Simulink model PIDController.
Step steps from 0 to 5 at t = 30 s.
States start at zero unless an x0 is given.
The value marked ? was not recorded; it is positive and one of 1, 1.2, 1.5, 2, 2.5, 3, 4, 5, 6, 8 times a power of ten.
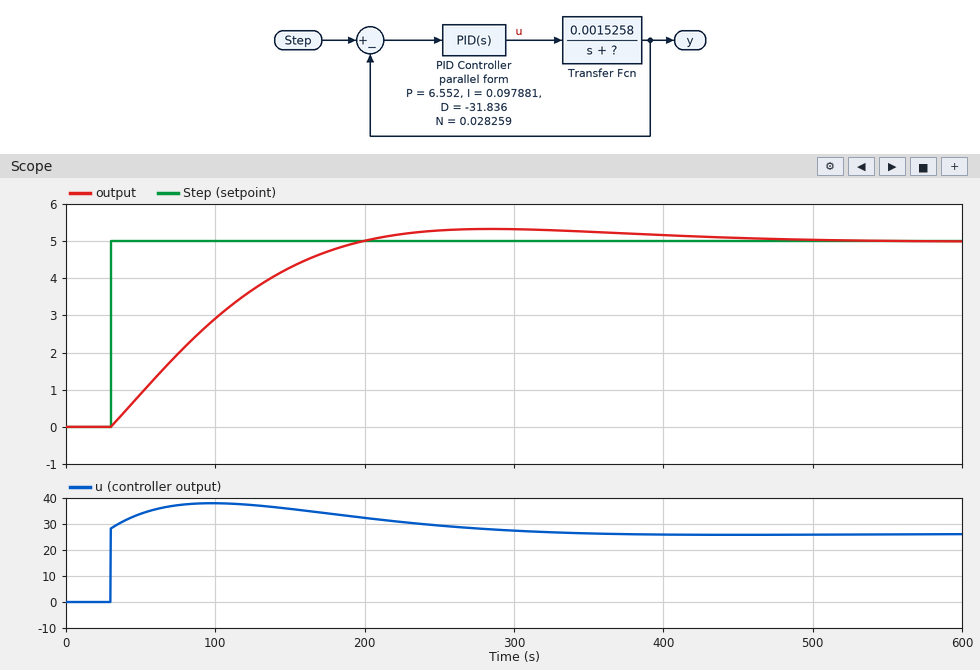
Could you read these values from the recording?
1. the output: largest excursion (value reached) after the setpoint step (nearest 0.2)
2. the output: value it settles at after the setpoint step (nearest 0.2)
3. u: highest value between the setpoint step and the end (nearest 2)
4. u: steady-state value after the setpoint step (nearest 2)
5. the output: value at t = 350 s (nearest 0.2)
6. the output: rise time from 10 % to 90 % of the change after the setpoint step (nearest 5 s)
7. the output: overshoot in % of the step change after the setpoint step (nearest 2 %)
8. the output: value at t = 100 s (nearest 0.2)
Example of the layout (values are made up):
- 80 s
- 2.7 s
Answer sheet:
- 5.4
- 5.0
- 38
- 26
- 5.2
- 120 s
- 6 %
- 3.0
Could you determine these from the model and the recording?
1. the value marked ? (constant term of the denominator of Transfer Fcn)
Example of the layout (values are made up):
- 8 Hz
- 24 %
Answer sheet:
- 0.008
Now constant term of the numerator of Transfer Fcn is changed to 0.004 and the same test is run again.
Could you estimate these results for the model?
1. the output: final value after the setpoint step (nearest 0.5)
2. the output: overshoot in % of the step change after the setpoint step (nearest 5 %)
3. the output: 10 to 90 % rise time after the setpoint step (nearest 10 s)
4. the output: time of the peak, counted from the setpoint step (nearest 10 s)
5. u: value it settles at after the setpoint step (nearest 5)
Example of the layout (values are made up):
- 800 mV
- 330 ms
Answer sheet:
- 5.0
- 10 %
- 60 s
- 130 s
- 10
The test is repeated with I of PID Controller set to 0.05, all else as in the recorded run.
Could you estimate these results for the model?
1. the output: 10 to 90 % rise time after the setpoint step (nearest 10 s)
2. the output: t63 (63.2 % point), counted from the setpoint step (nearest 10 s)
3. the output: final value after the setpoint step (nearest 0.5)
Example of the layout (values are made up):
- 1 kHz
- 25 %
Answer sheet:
- 220 s
- 100 s
- 5.0
